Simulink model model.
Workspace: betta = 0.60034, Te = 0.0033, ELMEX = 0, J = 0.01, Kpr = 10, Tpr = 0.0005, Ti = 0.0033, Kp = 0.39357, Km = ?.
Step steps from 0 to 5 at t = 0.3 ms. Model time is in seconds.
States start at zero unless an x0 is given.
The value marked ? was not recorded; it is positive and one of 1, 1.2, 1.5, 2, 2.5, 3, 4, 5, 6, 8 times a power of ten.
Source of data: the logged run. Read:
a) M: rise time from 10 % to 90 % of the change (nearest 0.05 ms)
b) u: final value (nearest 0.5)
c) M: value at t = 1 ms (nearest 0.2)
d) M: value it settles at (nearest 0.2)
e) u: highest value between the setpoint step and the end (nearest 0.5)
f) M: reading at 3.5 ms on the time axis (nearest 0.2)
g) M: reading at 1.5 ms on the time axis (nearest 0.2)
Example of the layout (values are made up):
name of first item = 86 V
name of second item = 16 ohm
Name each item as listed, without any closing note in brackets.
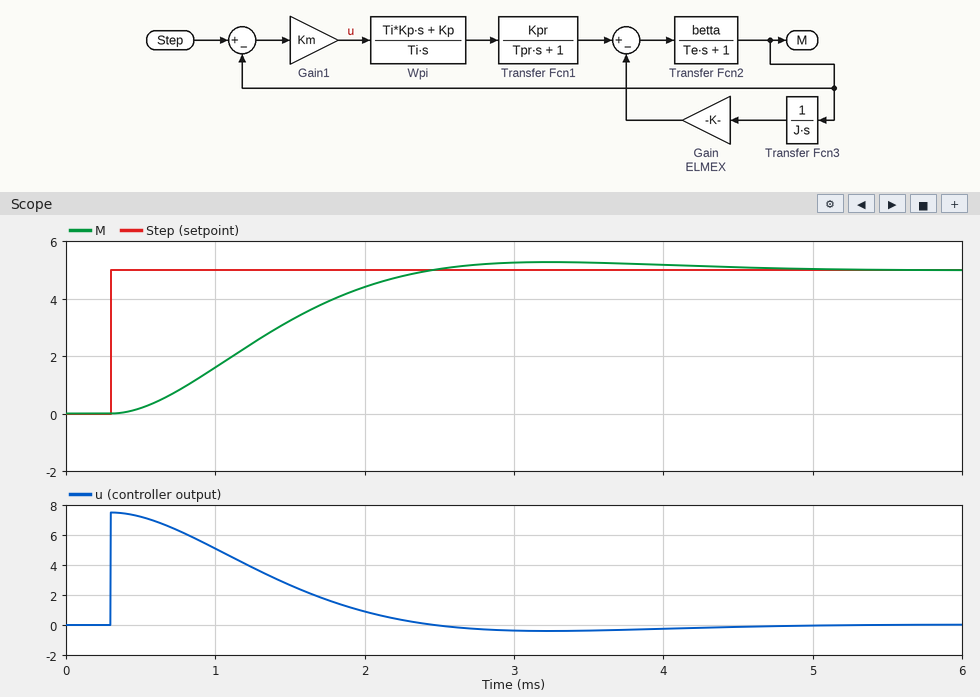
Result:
M: rise time from 10 % to 90 % of the change = 1.40 ms
u: final value = 0.0
M: value at t = 1 ms = 1.6
M: value it settles at = 5.0
u: highest value between the setpoint step and the end = 7.5
M: reading at 3.5 ms on the time axis = 5.2
M: reading at 1.5 ms on the time axis = 3.2
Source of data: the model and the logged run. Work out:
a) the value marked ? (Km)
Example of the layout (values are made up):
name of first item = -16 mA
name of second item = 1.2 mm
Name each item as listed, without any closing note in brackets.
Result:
the value marked ? = 1.5
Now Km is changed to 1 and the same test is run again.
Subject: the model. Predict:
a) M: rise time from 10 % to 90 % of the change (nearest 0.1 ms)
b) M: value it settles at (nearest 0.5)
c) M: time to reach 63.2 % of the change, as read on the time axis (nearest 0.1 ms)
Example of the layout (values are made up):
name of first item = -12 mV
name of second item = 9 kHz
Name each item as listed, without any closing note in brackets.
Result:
M: rise time from 10 % to 90 % of the change = 2.2 ms
M: value it settles at = 5.0
M: time to reach 63.2 % of the change, as read on the time axis = 1.9 ms
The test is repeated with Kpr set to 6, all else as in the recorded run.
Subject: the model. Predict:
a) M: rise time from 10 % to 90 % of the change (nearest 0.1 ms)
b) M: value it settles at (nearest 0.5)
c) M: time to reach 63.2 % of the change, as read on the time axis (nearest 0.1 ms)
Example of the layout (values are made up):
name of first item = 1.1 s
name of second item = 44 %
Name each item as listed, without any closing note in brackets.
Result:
M: rise time from 10 % to 90 % of the change = 2.5 ms
M: value it settles at = 5.0
M: time to reach 63.2 % of the change, as read on the time axis = 2.0 ms
